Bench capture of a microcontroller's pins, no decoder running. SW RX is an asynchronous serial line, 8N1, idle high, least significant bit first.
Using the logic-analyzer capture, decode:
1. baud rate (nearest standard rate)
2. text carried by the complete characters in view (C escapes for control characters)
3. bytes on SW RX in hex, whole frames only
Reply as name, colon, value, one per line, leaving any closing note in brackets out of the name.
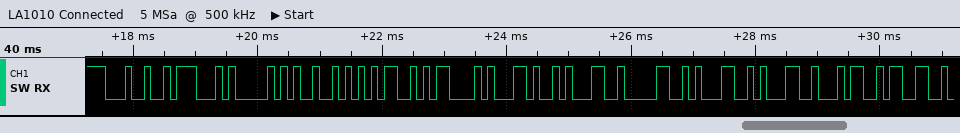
baud rate: 9600 baud
text carried by the complete characters in view: "$GPRMC,101143"
bytes on SW RX in hex, whole frames only: 24 47 50 52 4D 43 2C 31 30 31 31 34 33
